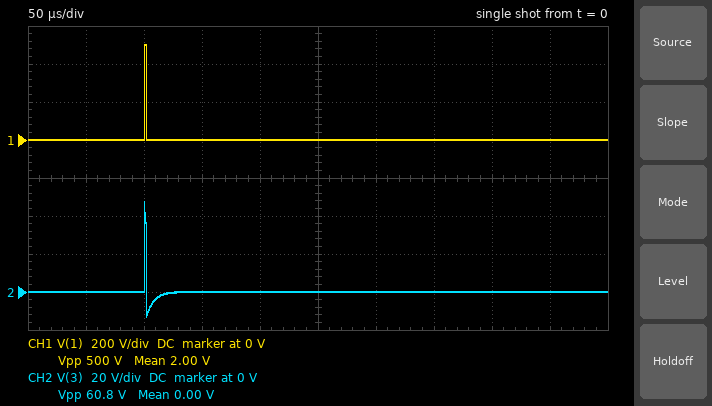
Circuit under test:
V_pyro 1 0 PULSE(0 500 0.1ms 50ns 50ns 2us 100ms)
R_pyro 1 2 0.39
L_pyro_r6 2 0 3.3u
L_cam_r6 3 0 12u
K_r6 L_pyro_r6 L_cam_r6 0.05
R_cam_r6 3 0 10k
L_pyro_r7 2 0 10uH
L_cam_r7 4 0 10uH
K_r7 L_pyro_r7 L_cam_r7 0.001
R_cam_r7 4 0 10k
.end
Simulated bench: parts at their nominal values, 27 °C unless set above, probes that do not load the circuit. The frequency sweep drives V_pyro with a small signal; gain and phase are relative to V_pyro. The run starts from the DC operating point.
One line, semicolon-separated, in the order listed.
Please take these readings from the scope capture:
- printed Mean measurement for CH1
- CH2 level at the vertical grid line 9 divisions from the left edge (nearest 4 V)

2.00 V; 0 V
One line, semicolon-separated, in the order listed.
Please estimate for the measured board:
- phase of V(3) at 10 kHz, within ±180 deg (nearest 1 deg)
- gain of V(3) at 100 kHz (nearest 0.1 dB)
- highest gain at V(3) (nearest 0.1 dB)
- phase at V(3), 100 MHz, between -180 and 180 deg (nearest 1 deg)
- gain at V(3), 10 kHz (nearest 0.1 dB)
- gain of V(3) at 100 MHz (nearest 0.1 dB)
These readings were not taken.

68 deg; -20.7 dB; -20.4 dB; -37 deg; -29.0 dB; -22.4 dB
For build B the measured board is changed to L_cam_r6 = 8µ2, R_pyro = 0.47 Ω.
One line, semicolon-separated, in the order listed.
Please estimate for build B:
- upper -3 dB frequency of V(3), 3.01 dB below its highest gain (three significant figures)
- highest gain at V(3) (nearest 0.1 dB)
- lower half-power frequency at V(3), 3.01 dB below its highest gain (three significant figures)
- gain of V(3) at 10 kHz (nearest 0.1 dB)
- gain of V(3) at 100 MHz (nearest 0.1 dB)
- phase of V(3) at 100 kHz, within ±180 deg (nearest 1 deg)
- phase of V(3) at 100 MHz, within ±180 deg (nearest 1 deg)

195 MHz; -22.1 dB; 30.1 kHz; -32.1 dB; -23.1 dB; 17 deg; -27 deg
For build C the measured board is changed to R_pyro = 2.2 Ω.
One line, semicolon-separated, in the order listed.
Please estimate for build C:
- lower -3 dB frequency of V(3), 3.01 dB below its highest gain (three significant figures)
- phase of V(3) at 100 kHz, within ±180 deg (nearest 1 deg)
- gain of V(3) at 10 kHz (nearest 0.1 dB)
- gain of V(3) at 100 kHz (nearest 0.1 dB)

141 kHz; 55 deg; -43.4 dB; -25.2 dB
